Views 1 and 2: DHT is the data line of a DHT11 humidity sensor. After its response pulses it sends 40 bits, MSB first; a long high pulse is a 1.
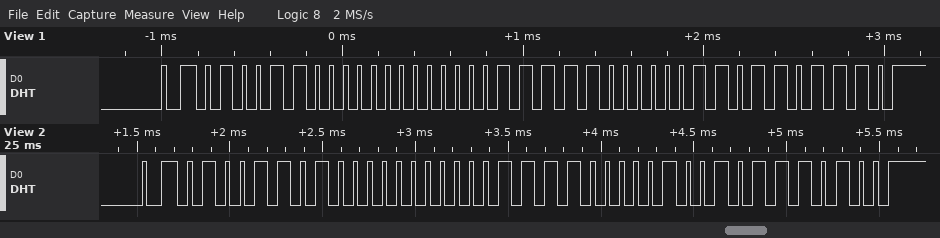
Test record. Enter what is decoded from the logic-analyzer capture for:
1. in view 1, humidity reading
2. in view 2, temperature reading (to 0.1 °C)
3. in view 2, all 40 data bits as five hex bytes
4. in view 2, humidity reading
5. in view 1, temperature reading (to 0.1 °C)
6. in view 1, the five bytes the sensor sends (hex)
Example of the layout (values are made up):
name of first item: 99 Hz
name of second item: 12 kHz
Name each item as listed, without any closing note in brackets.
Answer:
in view 1, humidity reading: 76 %
in view 2, temperature reading: 30.9 °C
in view 2, all 40 data bits as five hex bytes: 4D 00 1E 09 74
in view 2, humidity reading: 77 %
in view 1, temperature reading: 31.3 °C
in view 1, the five bytes the sensor sends: 4C 00 1F 03 6E
